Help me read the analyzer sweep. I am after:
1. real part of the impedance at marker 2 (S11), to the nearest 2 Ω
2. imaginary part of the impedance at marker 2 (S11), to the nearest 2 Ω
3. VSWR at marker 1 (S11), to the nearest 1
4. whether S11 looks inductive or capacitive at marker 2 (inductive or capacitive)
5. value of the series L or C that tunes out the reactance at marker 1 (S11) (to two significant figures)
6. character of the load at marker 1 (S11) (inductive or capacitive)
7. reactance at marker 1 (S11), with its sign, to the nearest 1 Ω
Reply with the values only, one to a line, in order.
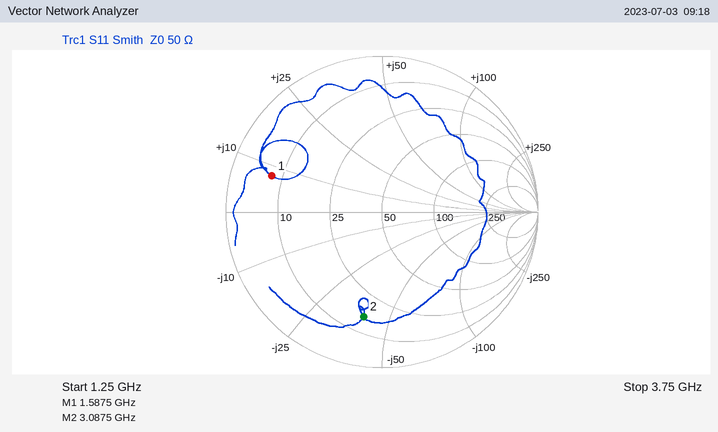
16 Ω
-40 Ω
7
capacitive
13 pF
inductive
+8 Ω
